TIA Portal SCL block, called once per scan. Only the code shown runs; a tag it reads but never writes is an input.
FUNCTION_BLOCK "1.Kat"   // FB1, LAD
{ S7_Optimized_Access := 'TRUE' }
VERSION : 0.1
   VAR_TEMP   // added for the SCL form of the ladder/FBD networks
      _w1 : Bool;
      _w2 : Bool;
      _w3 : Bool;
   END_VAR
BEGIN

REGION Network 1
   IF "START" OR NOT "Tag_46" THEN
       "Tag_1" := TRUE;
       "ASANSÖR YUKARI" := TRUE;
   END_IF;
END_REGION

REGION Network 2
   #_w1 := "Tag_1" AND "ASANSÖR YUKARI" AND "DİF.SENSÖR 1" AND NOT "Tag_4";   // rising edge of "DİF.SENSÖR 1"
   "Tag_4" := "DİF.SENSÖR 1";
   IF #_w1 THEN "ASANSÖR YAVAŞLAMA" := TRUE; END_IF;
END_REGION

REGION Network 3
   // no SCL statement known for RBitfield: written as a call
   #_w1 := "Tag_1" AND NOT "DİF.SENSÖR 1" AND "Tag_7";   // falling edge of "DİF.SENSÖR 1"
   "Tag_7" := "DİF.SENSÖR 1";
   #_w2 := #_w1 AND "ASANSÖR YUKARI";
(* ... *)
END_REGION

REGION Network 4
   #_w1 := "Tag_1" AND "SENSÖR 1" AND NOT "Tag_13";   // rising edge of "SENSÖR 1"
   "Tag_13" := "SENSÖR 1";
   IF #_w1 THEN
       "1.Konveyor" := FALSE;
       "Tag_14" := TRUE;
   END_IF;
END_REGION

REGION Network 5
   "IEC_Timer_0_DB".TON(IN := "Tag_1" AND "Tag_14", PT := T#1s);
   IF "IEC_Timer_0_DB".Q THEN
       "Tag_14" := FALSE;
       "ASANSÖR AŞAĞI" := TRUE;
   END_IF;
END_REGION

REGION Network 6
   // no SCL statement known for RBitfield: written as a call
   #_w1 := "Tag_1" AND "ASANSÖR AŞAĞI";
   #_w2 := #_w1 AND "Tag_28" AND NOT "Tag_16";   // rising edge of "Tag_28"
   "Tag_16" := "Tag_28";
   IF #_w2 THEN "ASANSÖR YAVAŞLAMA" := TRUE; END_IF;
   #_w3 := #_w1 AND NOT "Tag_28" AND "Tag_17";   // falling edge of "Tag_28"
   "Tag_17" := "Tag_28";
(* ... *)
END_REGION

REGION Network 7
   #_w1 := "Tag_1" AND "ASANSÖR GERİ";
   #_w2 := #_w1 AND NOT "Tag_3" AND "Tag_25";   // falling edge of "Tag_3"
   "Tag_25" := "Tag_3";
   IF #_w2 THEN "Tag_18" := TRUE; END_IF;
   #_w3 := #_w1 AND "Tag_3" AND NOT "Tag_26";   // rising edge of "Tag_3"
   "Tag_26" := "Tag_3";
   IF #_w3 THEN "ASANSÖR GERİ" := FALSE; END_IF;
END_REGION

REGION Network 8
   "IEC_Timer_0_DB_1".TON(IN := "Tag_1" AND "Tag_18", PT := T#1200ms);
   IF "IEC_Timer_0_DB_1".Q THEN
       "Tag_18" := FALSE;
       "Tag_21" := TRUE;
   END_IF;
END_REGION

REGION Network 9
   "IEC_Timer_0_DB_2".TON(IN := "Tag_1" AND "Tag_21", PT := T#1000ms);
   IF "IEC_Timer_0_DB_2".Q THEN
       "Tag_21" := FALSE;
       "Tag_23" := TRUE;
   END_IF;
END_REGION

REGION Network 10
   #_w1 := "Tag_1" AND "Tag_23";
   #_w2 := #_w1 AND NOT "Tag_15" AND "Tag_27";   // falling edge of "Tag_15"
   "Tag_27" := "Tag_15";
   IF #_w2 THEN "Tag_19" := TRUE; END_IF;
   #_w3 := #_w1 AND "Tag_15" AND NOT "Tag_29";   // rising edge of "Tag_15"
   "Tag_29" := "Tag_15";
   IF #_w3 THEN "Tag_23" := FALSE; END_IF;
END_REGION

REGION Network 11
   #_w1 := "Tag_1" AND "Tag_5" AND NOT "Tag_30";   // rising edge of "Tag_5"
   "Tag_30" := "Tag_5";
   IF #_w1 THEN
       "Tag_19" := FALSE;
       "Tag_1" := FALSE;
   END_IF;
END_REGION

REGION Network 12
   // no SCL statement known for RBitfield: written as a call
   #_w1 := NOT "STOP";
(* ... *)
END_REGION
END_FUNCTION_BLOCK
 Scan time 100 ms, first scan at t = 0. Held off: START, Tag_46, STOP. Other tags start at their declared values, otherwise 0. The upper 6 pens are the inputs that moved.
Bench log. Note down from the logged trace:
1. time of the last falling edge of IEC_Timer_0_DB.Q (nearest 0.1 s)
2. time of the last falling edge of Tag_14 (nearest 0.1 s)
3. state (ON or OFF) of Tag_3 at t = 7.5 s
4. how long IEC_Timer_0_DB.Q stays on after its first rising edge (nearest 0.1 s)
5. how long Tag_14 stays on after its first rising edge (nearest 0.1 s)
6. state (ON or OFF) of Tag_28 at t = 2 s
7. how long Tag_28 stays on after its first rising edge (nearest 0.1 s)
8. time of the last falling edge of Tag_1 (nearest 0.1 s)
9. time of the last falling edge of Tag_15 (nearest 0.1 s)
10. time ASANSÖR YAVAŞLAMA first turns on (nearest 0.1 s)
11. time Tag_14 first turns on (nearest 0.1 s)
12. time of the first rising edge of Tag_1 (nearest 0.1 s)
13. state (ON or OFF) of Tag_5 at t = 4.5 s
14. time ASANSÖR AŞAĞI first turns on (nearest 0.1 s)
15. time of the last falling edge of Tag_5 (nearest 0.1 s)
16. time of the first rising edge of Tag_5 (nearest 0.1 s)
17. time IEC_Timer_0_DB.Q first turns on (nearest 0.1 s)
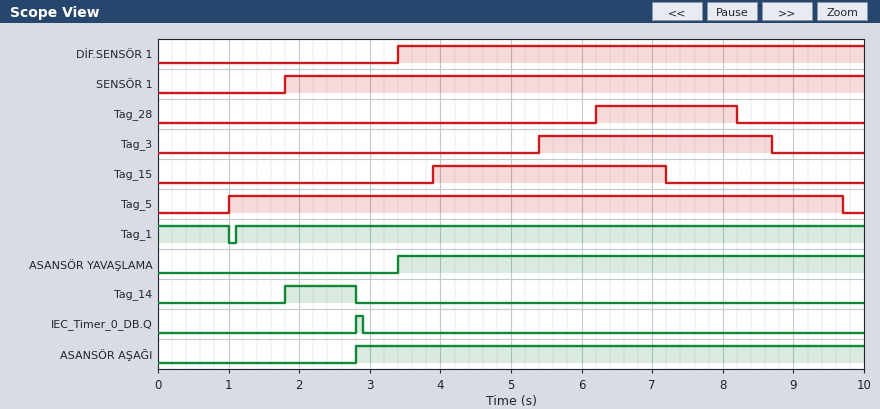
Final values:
2.9 s
2.8 s
ON
0.1 s
1.0 s
OFF
2.0 s
1.0 s
7.2 s
3.4 s
1.8 s
1.1 s
ON
2.8 s
9.7 s
1.0 s
2.8 s
